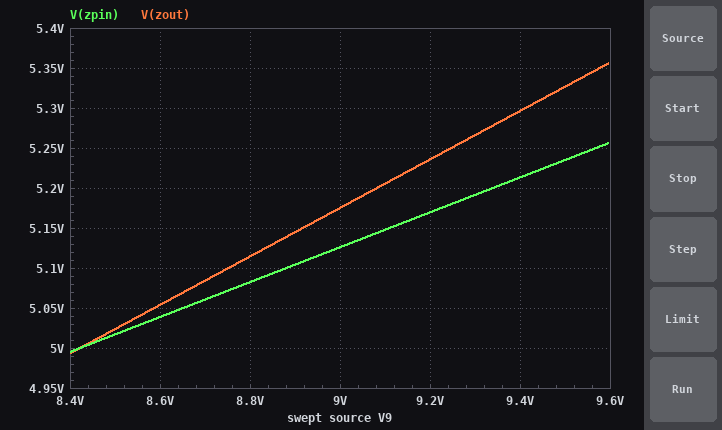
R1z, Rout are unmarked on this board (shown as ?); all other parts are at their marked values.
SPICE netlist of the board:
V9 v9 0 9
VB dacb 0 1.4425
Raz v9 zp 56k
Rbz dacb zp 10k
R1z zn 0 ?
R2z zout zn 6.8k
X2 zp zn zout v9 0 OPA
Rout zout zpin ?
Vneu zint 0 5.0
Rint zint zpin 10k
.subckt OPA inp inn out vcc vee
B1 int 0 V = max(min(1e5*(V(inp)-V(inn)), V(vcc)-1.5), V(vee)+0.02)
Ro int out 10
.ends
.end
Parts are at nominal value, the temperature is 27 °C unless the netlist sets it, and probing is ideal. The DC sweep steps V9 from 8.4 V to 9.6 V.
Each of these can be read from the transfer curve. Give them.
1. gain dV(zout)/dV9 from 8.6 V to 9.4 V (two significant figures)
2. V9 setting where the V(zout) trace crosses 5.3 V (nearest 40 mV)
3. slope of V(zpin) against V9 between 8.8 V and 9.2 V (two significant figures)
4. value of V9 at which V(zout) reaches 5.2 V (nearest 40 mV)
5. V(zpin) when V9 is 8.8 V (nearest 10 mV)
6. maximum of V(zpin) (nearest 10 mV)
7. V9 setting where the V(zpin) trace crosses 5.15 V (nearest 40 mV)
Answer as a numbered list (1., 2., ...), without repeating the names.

1. 0.30 V/V
2. 9.40 V
3. 0.22 V/V
4. 9.08 V
5. 5.08 V
6. 5.26 V
7. 9.12 V
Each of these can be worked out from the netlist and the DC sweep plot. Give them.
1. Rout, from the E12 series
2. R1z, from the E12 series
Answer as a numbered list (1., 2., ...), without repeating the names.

1. 3.9 kΩ
2. 6.8 kΩ
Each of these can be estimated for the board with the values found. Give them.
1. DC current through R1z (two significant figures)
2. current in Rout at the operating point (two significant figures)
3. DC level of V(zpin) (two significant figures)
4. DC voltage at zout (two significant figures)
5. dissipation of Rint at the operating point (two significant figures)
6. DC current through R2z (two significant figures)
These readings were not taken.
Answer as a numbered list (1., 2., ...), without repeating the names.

1. 380 µA
2. 13 µA
3. 5.1 V
4. 5.2 V
5. 1.6 µW
6. 380 µA
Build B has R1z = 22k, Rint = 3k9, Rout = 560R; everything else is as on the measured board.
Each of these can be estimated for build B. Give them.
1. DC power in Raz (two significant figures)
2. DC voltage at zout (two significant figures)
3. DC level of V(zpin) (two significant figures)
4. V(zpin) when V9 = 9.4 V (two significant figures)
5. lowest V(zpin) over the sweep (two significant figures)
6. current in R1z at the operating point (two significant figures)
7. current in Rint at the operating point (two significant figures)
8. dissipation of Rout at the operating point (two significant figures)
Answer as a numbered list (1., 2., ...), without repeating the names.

1. 730 µW
2. 3.4 V
3. 3.6 V
4. 3.7 V
5. 3.5 V
6. 120 µA
7. 360 µA
8. 73 µW
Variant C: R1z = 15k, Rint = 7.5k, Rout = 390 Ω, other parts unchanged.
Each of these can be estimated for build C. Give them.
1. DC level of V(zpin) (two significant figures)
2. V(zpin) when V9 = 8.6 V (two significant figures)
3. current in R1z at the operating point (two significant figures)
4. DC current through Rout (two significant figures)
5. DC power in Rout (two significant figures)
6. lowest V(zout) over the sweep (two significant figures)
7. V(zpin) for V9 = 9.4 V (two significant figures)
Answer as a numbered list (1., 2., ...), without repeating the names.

1. 3.8 V
2. 3.7 V
3. 170 µA
4. 160 µA
5. 9.6 µW
6. 3.6 V
7. 3.9 V
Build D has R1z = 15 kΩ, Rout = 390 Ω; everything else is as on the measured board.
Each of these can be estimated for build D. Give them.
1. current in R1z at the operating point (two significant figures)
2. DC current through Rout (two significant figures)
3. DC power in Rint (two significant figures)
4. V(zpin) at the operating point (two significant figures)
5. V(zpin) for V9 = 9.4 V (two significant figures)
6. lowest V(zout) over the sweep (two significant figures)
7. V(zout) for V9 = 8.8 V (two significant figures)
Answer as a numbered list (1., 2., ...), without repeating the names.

1. 170 µA
2. 120 µA
3. 140 µW
4. 3.8 V
5. 3.9 V
6. 3.6 V
7. 3.7 V
